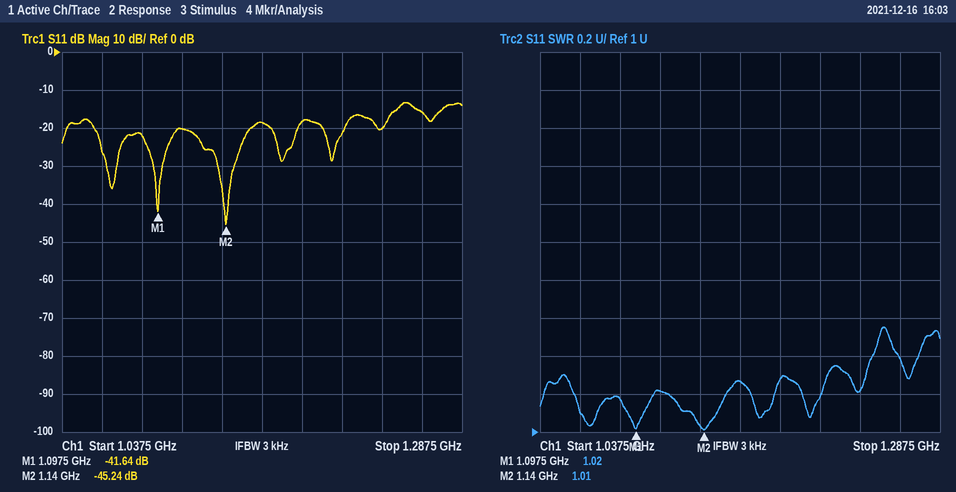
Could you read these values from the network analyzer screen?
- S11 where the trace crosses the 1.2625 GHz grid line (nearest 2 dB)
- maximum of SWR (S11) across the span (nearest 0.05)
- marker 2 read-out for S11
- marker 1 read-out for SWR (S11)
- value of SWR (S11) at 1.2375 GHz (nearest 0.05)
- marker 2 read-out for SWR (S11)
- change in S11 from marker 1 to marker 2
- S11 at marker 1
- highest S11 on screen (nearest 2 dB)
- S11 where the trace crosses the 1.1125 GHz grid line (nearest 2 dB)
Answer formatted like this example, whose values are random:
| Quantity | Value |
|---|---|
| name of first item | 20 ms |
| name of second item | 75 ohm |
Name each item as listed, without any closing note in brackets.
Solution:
| Quantity | Value |
|---|---|
| S11 where the trace crosses the 1.2625 GHz grid line | -16 dB |
| maximum of SWR (S11) across the span | 1.55 |
| marker 2 read-out for S11 | -45.24 dB |
| marker 1 read-out for SWR | 1.02 |
| value of SWR (S11) at 1.2375 GHz | 1.20 |
| marker 2 read-out for SWR | 1.01 |
| change in S11 from marker 1 to marker 2 | -3.60 dB |
| S11 at marker 1 | -41.64 dB |
| highest S11 on screen | -14 dB |
| S11 where the trace crosses the 1.1125 GHz grid line | -20 dB |
